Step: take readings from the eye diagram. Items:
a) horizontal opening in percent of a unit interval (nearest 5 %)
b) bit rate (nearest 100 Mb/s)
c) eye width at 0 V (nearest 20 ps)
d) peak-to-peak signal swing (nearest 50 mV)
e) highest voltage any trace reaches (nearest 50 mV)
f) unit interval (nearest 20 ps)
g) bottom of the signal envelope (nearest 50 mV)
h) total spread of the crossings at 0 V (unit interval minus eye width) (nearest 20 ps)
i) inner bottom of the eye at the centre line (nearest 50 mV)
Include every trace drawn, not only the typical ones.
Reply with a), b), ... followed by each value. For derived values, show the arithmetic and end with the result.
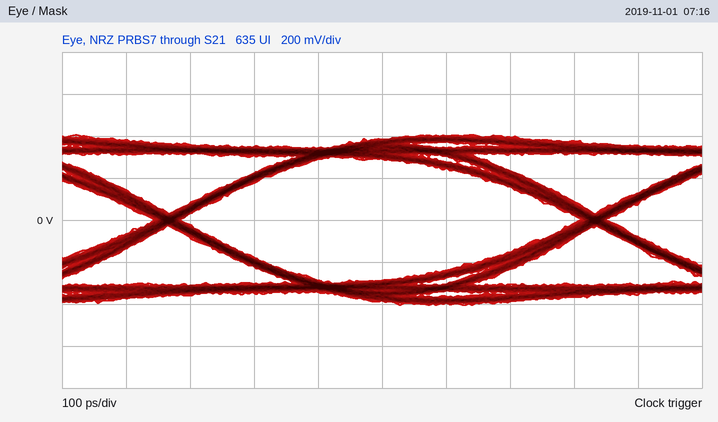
a) 620 ps / 660 ps ≈ 93.9 %, so 95 % to the nearest 5 %
b) 1.5 Gb/s
c) 620 ps
d) 800 mV
e) 400 mV
f) 660 ps
g) -400 mV
h) 40 ps
i) -300 mV
